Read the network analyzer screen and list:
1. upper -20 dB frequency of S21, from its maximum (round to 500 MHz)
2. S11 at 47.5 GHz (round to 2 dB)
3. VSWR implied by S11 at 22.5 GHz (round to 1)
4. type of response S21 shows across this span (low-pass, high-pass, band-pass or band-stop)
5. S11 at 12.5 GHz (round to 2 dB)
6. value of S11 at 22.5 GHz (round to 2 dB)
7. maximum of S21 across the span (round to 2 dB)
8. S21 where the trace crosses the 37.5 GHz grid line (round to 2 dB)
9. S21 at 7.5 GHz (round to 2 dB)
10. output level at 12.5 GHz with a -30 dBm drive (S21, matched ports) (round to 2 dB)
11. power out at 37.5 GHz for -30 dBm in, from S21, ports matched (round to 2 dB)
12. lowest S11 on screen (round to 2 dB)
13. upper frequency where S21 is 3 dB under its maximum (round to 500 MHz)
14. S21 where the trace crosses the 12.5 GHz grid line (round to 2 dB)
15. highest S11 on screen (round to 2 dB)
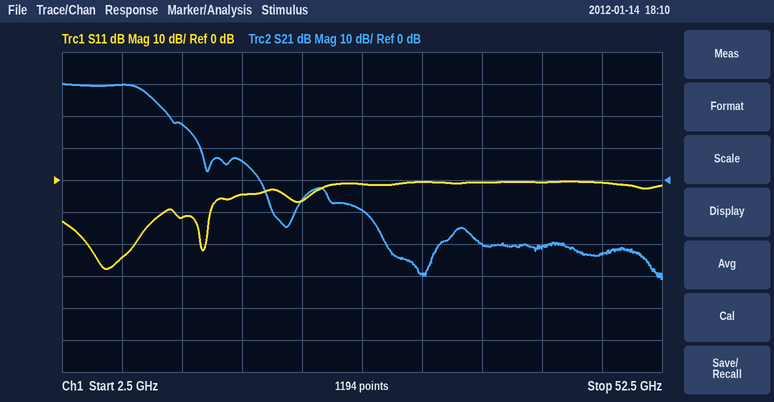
14.0 GHz
0 dB
3
low-pass
-12 dB
-6 dB
30 dB
-20 dB
30 dB
-12 dBm
-50 dBm
-28 dB
9.5 GHz
18 dB
0 dB
